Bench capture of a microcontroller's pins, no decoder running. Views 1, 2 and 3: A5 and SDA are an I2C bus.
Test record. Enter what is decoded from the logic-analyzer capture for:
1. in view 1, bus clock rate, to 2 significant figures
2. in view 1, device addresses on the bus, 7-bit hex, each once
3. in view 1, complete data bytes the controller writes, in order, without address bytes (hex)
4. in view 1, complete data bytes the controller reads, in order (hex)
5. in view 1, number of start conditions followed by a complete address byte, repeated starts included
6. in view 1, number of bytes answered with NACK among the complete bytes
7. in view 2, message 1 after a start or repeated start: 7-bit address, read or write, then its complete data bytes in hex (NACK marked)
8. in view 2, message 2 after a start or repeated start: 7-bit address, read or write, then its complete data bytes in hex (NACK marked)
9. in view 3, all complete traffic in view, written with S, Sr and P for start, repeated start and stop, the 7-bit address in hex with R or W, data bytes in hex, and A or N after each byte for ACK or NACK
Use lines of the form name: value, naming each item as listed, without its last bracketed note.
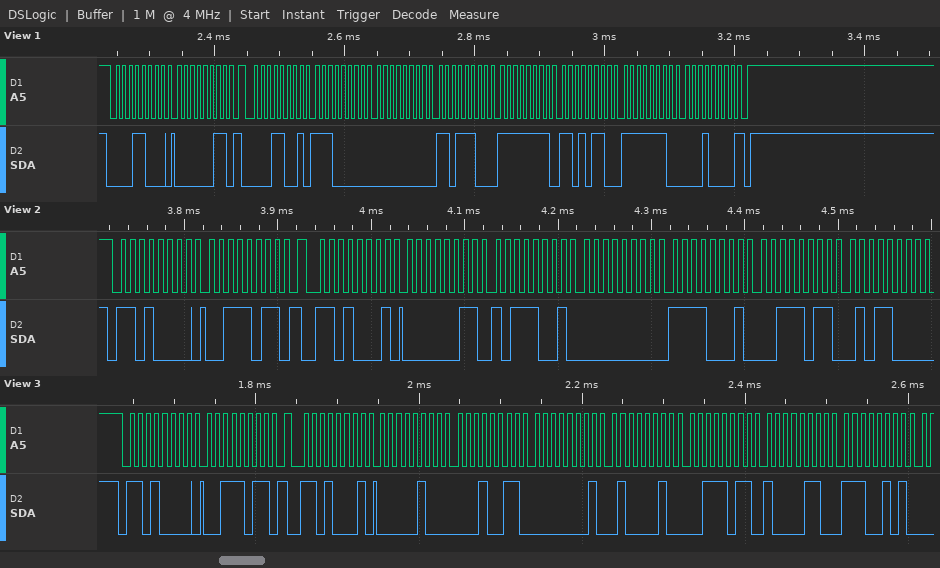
in view 1, bus clock rate, to 2 significant figures: 100 kHz
in view 1, device addresses on the bus, 7-bit hex, each once: 0x0C
in view 1, complete data bytes the controller writes, in order, without address bytes: 03
in view 1, complete data bytes the controller reads, in order: E0 00 DC FF D6 FE 10
in view 1, number of start conditions followed by a complete address byte, repeated starts included: 2
in view 1, number of bytes answered with NACK among the complete bytes: 1
in view 2, message 1 after a start or repeated start: 7-bit address, read or write, then its complete data bytes in hex: 0x68 write: 3B
in view 2, message 2 after a start or repeated start: 7-bit address, read or write, then its complete data bytes in hex: 0x68 read: 03 B9 00 F1 3B 58
in view 3, all complete traffic in view, written with S, Sr and P for start, repeated start and stop, the 7-bit address in hex with R or W, data bytes in hex, and A or N after each byte for ACK or NACK: S 68W A 3B A Sr 68R A 04 A 13 A 01 A 42 A 3B A 86 A E5 A
